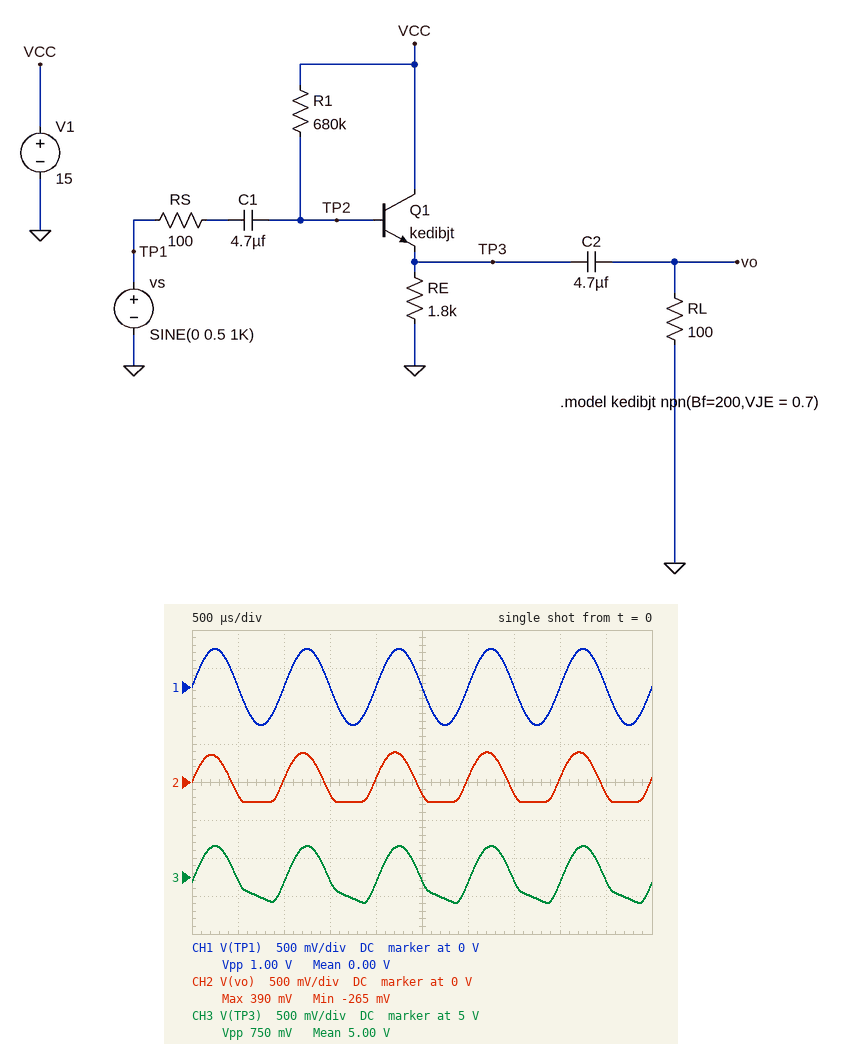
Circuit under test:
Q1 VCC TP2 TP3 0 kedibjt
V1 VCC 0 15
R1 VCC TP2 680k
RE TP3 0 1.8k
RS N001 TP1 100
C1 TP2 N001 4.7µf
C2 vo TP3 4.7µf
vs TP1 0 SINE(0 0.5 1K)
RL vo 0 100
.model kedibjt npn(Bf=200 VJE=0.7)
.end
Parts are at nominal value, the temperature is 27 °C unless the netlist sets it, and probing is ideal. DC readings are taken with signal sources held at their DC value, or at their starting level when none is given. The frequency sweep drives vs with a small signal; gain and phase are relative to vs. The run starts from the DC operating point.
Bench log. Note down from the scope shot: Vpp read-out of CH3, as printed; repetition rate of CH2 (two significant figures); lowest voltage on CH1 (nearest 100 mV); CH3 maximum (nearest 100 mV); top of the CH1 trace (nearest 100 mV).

750 mV
1.0 kHz
-500 mV
5.4 V
500 mV
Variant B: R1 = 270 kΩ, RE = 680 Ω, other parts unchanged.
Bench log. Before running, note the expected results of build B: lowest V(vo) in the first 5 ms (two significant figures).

-470 mV
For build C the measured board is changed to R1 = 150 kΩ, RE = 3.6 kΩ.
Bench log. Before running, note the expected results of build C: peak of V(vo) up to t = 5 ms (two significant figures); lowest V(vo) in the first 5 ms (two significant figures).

420 mV
-320 mV
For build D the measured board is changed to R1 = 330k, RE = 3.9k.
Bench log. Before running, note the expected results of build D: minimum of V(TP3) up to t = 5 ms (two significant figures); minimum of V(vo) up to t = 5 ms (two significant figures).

9.7 V
-250 mV
